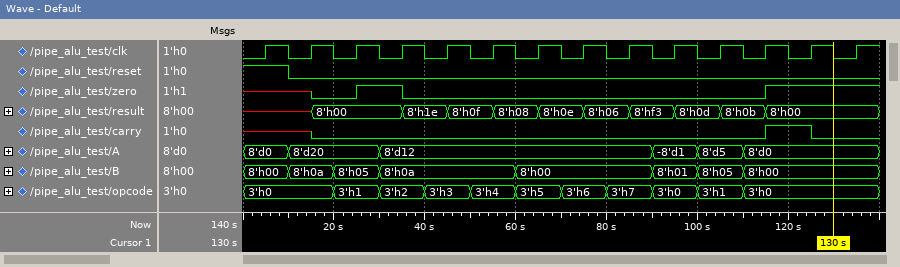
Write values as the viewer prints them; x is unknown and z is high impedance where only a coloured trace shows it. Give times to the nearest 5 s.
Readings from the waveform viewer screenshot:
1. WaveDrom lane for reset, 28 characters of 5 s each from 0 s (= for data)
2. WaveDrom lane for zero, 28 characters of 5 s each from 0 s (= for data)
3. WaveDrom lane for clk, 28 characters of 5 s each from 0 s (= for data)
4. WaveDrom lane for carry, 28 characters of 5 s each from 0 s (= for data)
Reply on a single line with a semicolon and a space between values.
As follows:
{name: 'reset', wave: '1.0.........................'}; {name: 'zero', wave: 'x..0.1.0...............1....'}; {name: 'clk', wave: '0101010101010101010101010101'}; {name: 'carry', wave: 'x..0...................1.0..'}
